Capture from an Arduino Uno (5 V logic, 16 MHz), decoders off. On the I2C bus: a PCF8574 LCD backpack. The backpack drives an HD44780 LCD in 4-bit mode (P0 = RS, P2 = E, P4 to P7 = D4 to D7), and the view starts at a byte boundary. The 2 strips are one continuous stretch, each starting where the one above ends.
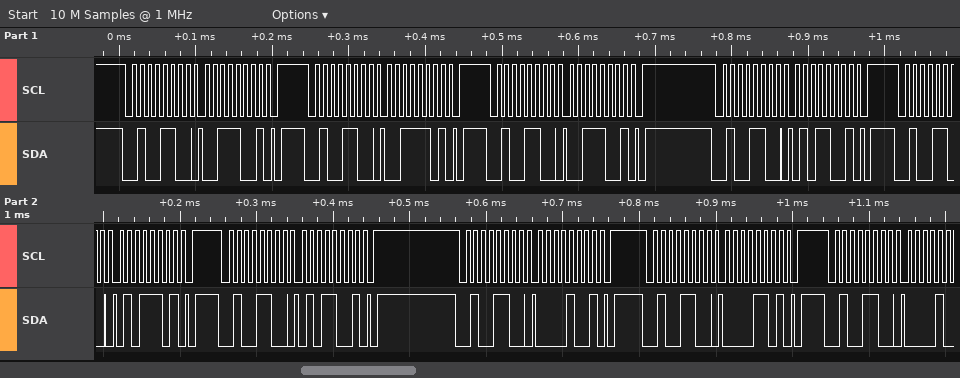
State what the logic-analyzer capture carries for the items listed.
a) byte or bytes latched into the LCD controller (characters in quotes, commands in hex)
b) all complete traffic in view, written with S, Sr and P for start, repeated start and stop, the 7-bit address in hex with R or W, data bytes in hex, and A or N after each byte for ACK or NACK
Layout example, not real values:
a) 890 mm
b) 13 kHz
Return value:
a) '5'
b) S 26W A 39 A P S 26W A 3D A P S 26W A 39 A P S 26W A 59 A P S 26W A 5D A P S 26W A 59 A P S 26W A 09 A P S 26W A 0D A P S 26W A
